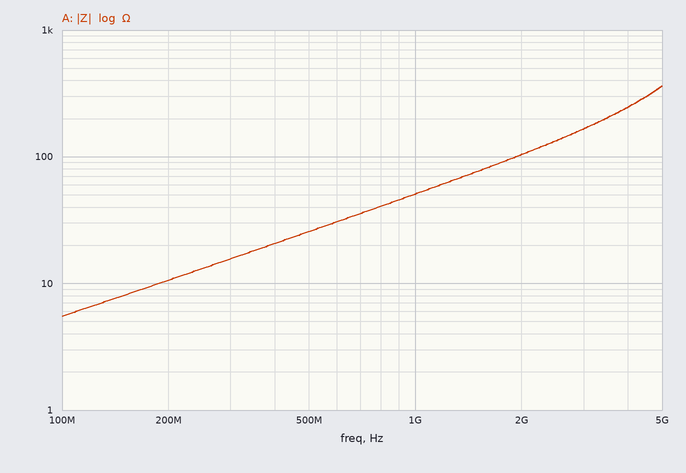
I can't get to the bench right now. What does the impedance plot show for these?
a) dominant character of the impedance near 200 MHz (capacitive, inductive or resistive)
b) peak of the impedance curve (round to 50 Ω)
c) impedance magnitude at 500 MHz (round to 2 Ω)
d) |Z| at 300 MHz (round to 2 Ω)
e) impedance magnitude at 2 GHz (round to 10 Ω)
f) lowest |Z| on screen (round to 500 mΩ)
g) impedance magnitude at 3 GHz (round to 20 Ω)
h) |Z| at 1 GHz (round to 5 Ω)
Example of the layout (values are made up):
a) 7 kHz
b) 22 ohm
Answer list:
a) inductive
b) 350 Ω
c) 26 Ω
d) 16 Ω
e) 100 Ω
f) 5.5 Ω
g) 160 Ω
h) 50 Ω
